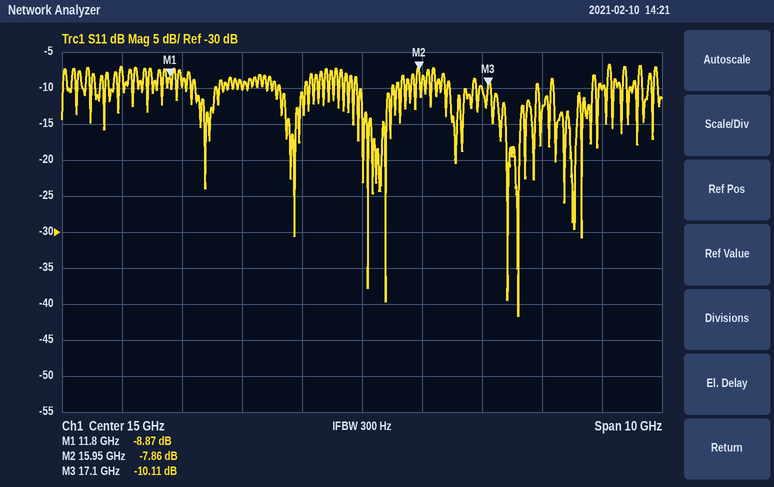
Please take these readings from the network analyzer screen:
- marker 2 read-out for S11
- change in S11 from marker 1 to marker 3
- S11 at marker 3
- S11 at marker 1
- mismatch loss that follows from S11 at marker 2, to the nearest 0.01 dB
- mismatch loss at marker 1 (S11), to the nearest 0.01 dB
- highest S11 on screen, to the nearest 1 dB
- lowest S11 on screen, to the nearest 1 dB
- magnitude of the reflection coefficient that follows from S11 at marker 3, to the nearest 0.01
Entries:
-7.86 dB
-1.24 dB
-10.11 dB
-8.87 dB
0.78 dB
0.60 dB
-7 dB
-42 dB
0.31
